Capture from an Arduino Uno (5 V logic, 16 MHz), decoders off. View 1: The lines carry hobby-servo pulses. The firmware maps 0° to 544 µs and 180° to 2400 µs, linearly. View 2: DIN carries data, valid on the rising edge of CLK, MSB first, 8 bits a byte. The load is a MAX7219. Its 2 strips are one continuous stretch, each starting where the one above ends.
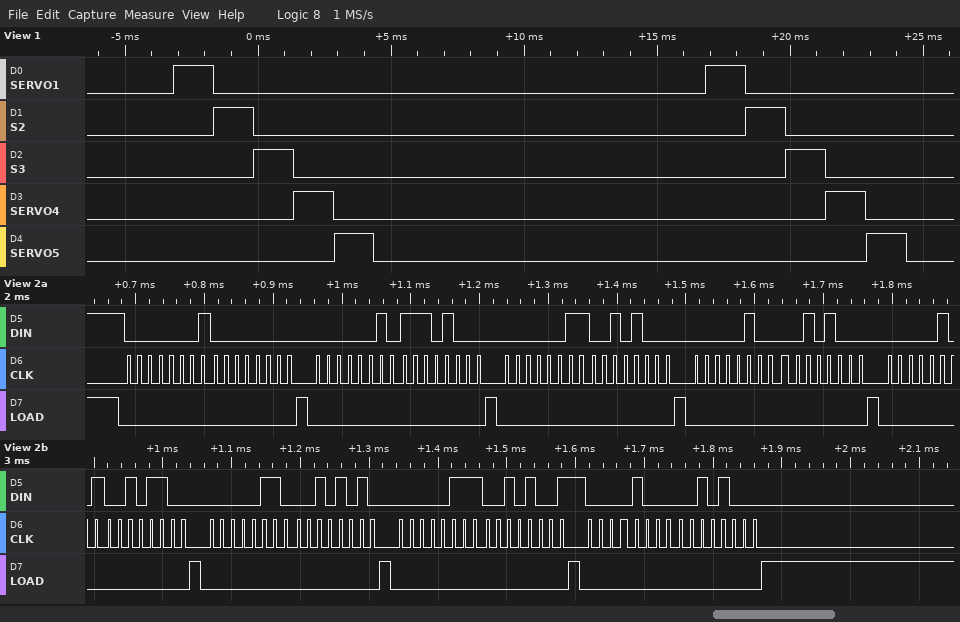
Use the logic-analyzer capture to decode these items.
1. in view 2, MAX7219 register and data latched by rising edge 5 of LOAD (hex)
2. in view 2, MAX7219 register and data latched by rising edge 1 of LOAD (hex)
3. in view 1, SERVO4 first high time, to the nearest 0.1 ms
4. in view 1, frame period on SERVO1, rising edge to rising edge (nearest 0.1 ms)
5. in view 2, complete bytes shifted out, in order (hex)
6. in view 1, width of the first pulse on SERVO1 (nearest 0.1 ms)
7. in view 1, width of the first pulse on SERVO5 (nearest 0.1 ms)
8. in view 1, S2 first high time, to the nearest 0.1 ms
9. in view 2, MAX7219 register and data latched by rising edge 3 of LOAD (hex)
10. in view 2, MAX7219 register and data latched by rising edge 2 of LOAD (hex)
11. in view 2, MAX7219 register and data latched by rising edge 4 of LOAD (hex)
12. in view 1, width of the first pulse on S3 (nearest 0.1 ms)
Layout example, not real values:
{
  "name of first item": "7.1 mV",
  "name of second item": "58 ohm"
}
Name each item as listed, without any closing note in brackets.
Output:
{
  "in view 2, MAX7219 register and data latched by rising edge 5 of LOAD": "register 0x5, data 0x2C",
  "in view 2, MAX7219 register and data latched by rising edge 1 of LOAD": "register 0x1, data 0x00",
  "in view 1, SERVO4 first high time, to the nearest 0.1 ms": "1.5 ms",
  "in view 1, frame period on SERVO1, rising edge to rising edge": "20.0 ms",
  "in view 2, complete bytes shifted out, in order": "01 00 02 E8 03 28 04 28 05 2C 06 2A 07 29 08 28",
  "in view 1, width of the first pulse on SERVO1": "1.5 ms",
  "in view 1, width of the first pulse on SERVO5": "1.5 ms",
  "in view 1, S2 first high time, to the nearest 0.1 ms": "1.5 ms",
  "in view 2, MAX7219 register and data latched by rising edge 3 of LOAD": "register 0x3, data 0x28",
  "in view 2, MAX7219 register and data latched by rising edge 2 of LOAD": "register 0x2, data 0xE8",
  "in view 2, MAX7219 register and data latched by rising edge 4 of LOAD": "register 0x4, data 0x28",
  "in view 1, width of the first pulse on S3": "1.5 ms"
}
